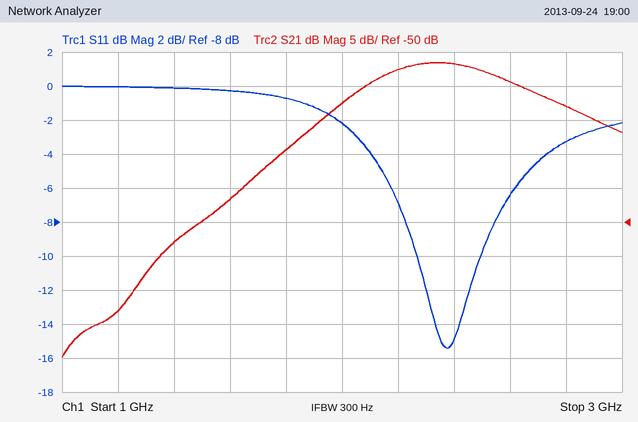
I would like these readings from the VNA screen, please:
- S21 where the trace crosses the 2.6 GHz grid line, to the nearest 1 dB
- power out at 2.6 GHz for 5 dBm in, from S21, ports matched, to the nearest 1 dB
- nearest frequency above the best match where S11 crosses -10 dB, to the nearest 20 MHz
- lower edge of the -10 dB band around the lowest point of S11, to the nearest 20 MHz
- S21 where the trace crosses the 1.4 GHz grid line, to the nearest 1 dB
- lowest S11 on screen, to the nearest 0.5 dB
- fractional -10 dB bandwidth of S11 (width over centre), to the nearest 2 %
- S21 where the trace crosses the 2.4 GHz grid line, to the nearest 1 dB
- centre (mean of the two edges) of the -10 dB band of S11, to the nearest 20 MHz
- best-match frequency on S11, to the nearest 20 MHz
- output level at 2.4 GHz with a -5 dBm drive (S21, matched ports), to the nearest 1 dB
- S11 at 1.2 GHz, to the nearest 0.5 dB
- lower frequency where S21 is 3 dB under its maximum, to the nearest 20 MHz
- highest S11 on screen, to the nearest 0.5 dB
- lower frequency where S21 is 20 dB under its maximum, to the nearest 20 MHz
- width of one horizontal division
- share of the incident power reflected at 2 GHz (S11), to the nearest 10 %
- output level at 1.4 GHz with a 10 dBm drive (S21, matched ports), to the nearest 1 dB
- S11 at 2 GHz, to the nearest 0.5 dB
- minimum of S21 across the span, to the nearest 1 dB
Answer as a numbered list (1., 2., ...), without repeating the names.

1. -29 dB
2. -24 dBm
3. 2.50 GHz
4. 2.26 GHz
5. -53 dB
6. -15.5 dB
7. 10 %
8. -27 dB
9. 2.38 GHz
10. 2.38 GHz
11. -32 dBm
12. 0.0 dB
13. 2.10 GHz
14. 0.0 dB
15. 1.60 GHz
16. 200 MHz
17. 60 %
18. -43 dBm
19. -2.0 dB
20. -70 dB
